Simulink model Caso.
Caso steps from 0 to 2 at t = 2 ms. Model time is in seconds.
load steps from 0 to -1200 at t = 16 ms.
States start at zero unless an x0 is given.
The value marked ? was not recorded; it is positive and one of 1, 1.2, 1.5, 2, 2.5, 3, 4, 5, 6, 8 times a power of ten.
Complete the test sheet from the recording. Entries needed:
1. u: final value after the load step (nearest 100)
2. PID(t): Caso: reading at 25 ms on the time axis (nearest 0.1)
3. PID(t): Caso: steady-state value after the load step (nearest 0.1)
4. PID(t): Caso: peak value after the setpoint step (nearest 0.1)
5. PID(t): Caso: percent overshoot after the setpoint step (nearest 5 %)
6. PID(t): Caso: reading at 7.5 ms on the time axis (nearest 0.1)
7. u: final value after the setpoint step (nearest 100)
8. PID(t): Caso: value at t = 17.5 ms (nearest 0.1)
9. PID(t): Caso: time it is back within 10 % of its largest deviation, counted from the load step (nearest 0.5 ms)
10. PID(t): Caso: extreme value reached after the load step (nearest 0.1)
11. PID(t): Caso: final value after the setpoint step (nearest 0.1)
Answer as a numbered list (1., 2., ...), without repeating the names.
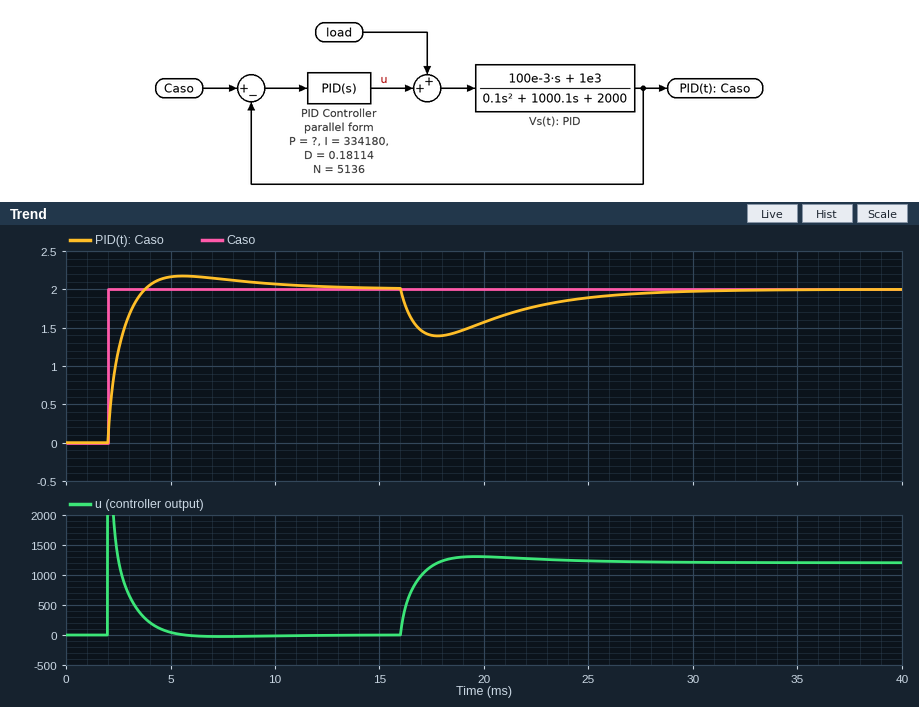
1. 1200
2. 1.9
3. 2.0
4. 2.2
5. 10 %
6. 2.1
7. 0
8. 1.4
9. 11.0 ms
10. 1.4
11. 2.0
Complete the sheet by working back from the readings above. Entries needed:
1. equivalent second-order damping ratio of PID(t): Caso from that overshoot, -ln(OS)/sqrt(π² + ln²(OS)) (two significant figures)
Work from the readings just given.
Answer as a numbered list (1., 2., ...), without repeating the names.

1. 0.59
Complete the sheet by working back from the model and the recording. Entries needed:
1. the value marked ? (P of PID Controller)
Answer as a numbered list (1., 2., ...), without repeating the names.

1. 1500
